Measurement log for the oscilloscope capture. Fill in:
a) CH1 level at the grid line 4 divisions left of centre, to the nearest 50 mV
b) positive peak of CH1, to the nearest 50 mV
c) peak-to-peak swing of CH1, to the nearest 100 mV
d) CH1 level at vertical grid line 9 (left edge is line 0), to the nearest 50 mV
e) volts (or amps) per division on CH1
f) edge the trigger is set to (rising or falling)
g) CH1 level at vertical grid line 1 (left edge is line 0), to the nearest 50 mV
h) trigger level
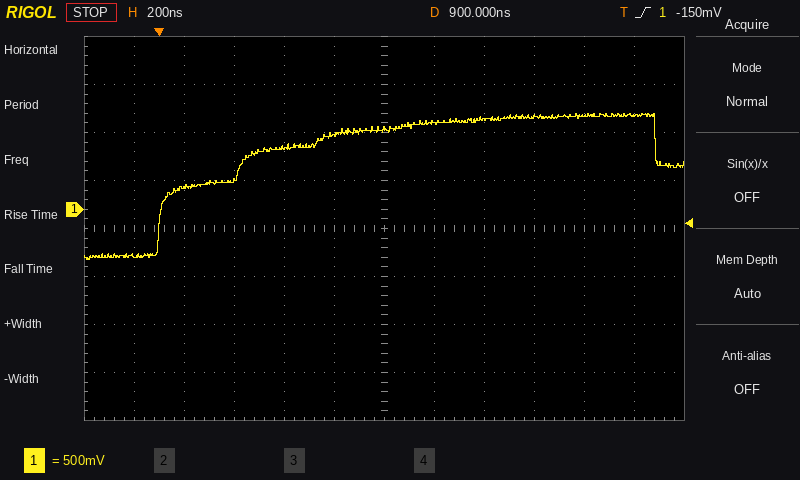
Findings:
250 mV
1.00 V
1.50 V
950 mV
500 mV
rising
-500 mV
-150 mV
